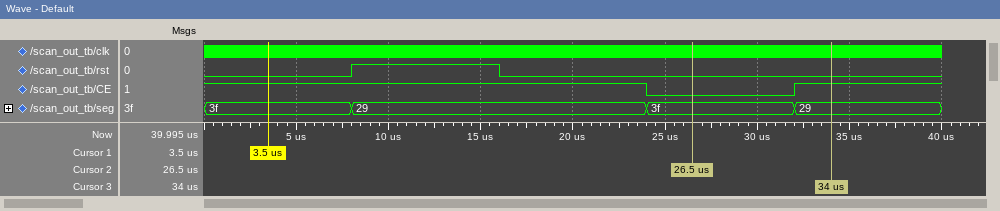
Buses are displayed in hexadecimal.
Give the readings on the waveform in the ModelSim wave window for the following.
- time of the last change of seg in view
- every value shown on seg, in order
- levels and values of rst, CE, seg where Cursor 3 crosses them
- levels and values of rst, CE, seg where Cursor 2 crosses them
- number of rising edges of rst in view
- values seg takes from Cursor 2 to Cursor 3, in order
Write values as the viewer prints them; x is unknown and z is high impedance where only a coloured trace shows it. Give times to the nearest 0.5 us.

32 us
3f, 29, 3f, 29
rst=0, CE=1, seg=29
rst=0, CE=0, seg=3f
1
3f, 29
